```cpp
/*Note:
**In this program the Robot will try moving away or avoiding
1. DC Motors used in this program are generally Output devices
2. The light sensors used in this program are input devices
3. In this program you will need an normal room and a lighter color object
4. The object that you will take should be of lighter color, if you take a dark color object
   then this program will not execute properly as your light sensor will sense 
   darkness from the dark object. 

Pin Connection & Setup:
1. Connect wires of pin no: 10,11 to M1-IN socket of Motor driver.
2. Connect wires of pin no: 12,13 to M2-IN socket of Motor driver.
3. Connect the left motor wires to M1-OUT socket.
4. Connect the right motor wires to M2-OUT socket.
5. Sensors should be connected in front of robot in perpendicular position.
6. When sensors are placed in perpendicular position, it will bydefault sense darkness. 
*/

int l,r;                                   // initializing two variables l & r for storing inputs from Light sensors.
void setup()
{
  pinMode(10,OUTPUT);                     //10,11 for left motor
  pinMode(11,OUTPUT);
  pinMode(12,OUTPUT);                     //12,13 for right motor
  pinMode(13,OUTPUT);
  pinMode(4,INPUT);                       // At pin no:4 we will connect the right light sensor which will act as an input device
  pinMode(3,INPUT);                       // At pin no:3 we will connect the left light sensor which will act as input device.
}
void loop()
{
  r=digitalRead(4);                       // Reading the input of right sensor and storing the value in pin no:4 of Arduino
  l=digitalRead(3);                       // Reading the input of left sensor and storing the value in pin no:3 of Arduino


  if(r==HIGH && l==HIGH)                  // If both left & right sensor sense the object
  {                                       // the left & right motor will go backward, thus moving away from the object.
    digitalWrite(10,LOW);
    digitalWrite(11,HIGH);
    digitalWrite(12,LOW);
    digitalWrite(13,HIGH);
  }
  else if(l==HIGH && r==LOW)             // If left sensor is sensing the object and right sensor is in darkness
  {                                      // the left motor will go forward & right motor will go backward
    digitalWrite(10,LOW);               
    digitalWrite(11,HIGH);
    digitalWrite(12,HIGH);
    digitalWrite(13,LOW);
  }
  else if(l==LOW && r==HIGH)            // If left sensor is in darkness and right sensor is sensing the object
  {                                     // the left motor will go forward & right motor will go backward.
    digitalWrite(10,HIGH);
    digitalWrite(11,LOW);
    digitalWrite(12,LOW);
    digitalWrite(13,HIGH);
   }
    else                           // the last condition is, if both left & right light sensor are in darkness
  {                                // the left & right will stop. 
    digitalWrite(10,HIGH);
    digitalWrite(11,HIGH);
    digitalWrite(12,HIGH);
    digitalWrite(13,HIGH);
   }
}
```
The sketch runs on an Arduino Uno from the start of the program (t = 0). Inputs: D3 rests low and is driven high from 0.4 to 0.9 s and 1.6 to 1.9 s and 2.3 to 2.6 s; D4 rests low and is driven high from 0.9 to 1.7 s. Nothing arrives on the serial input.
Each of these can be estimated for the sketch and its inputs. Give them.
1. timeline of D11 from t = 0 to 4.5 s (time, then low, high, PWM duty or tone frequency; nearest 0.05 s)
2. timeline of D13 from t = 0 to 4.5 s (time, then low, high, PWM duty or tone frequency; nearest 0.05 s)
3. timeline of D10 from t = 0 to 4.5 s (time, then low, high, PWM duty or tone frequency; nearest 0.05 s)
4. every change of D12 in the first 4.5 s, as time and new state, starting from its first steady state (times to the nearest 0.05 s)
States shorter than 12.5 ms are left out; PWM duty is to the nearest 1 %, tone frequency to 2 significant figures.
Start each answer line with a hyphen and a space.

- 0 s high; 0.9 s low; 1.6 s high
- 0 s high; 0.4 s low; 0.9 s high; 1.7 s low; 1.9 s high; 2.3 s low; 2.6 s high
- 0 s high; 0.4 s low; 0.9 s high; 1.6 s low; 1.9 s high; 2.3 s low; 2.6 s high
- 0 s high; 0.9 s low; 1.7 s high
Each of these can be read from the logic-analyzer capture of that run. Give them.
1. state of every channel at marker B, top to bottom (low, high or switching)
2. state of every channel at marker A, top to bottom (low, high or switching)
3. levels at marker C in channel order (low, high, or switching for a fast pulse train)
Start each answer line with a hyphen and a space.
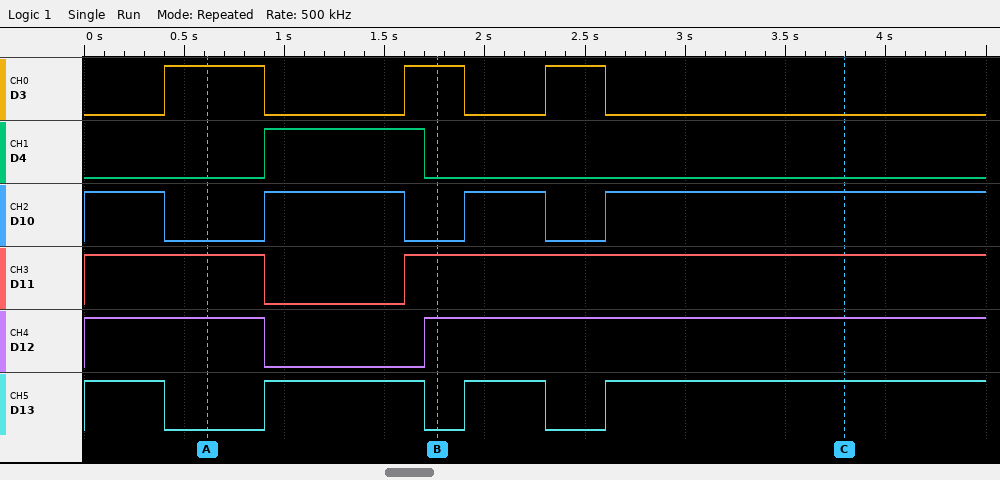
- D3 high, D4 low, D10 low, D11 high, D12 high, D13 low
- D3 high, D4 low, D10 low, D11 high, D12 high, D13 low
- D3 low, D4 low, D10 high, D11 high, D12 high, D13 high
